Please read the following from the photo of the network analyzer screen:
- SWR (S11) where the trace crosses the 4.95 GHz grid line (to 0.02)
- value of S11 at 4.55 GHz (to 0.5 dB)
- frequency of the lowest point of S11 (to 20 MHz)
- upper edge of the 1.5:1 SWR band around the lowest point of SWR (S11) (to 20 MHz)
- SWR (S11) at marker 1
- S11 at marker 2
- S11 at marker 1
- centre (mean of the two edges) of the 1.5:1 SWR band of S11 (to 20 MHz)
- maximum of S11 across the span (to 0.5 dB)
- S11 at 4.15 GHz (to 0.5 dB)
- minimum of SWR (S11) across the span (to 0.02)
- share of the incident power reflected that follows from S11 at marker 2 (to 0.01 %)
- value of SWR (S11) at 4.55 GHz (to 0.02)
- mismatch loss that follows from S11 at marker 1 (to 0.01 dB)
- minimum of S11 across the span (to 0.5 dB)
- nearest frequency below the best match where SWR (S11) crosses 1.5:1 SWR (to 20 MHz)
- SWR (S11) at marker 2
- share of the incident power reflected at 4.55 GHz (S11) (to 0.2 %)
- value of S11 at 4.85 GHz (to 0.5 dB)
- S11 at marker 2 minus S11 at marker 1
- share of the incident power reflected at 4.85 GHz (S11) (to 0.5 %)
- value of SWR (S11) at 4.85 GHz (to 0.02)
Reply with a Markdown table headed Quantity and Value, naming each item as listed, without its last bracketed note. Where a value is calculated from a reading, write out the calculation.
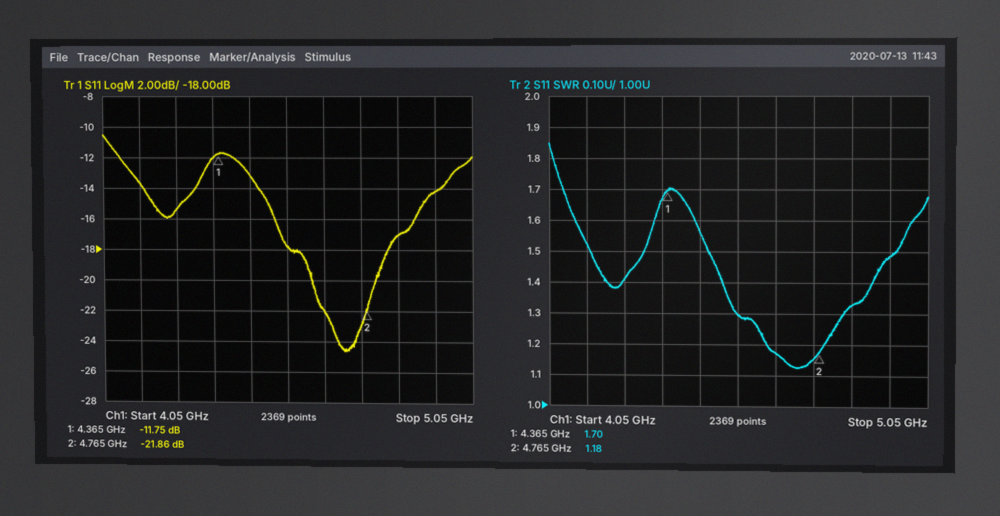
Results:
| Quantity | Value |
|---|---|
| SWR (S11) where the trace crosses the 4.95 GHz grid line | 1.48 |
| value of S11 at 4.55 GHz | -18.0 dB |
| frequency of the lowest point of S11 | 4.70 GHz |
| upper edge of the 1.5:1 SWR band around the lowest point of SWR (S11) | 4.96 GHz |
| SWR (S11) at marker 1 | 1.70 |
| S11 at marker 2 | -21.86 dB |
| S11 at marker 1 | -11.75 dB |
| centre (mean of the two edges) of the 1.5:1 SWR band of S11 | 4.72 GHz |
| maximum of S11 across the span | -10.5 dB |
| S11 at 4.15 GHz | -13.5 dB |
| minimum of SWR (S11) across the span | 1.12 |
| share of the incident power reflected that follows from S11 at marker 2 | 10^(-21.86/10) ≈ 0.65 % |
| value of SWR (S11) at 4.55 GHz | 1.30 |
| mismatch loss that follows from S11 at marker 1 | −10 log10(1 − 10^(-11.75/10)) ≈ 0.30 dB |
| minimum of S11 across the span | -24.5 dB |
| nearest frequency below the best match where SWR (S11) crosses 1.5:1 SWR | 4.48 GHz |
| SWR (S11) at marker 2 | 1.18 |
| share of the incident power reflected at 4.55 GHz (S11) | 10^(-18/10) ≈ 1.6 % |
| value of S11 at 4.85 GHz | -17.0 dB |
| S11 at marker 2 minus S11 at marker 1 | -21.86 − (-11.75) = -10.11 dB |
| share of the incident power reflected at 4.85 GHz (S11) | 10^(-17/10) ≈ 2.0 % |
| value of SWR (S11) at 4.85 GHz | 1.32 |
